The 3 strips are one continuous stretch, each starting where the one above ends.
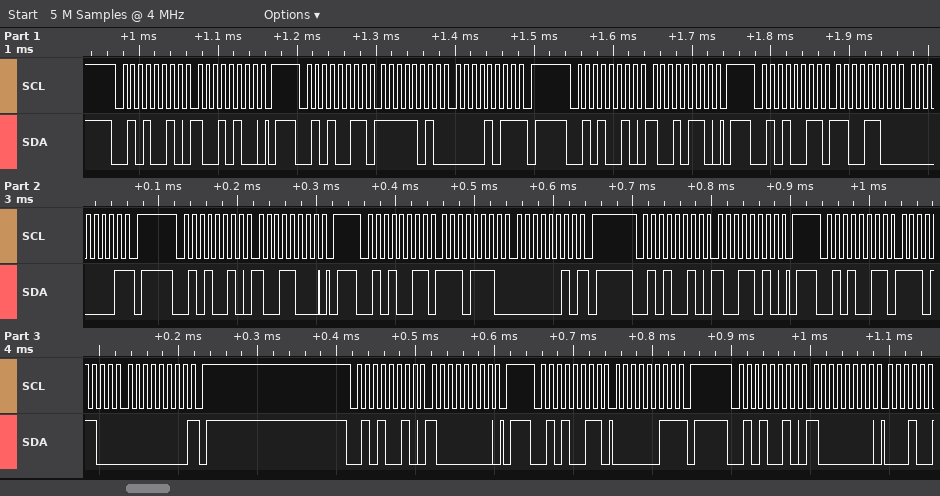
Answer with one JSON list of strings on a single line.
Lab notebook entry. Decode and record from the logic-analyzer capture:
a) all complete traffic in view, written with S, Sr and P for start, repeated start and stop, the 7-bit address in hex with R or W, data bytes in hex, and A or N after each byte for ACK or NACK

["S 29W A 94 A P S 29R A FA A 0B N P S 29W A 96 A P S 29R A CC A 01 N P S 29W A 98 A P S 29R A EE A 02 N P S 29W A 9A A P S 29R A EC A 00 N P S 29W A 80 A P S 29R A 03 N P S 29W A 80 A"]
